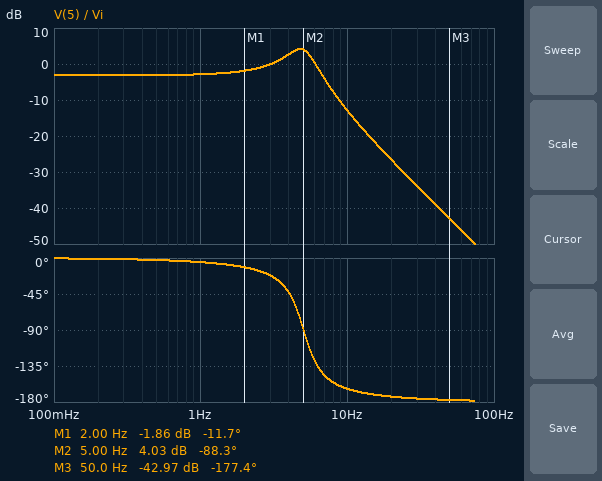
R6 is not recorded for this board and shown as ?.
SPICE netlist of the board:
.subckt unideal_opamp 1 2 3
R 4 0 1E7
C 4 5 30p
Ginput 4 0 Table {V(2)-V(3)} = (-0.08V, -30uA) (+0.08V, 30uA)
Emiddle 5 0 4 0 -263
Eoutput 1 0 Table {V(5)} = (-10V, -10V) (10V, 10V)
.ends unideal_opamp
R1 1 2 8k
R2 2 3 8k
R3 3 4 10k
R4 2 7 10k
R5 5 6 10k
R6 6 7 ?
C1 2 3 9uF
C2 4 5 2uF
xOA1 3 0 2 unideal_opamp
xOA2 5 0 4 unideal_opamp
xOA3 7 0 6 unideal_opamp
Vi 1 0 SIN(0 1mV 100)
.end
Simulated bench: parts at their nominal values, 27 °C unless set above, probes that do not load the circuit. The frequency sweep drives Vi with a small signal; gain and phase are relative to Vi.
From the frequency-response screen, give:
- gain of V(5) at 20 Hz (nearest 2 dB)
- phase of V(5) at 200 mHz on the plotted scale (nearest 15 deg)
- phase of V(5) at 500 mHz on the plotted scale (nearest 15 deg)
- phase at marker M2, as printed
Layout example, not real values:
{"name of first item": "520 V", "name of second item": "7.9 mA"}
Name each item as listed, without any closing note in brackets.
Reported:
{"gain of V(5) at 20 Hz": "-26 dB", "phase of V(5) at 200 mHz on the plotted scale": "0 deg", "phase of V(5) at 500 mHz on the plotted scale": "0 deg", "phase at marker M2, as printed": "-88.3 deg"}
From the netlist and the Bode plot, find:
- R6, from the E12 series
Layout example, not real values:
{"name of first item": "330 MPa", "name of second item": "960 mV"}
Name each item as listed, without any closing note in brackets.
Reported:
{"R6, from the E12 series": "18 kΩ"}
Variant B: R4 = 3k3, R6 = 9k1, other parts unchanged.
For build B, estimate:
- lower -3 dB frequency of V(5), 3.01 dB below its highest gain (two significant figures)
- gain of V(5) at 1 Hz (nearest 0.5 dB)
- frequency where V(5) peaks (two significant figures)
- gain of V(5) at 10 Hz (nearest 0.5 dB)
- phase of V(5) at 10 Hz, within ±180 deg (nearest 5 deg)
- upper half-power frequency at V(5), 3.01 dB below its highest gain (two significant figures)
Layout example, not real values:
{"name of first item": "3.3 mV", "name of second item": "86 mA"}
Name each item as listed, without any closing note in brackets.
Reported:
{"lower -3 dB frequency of V(5), 3.01 dB below its highest gain": "4.8 Hz", "gain of V(5) at 1 Hz": "-6.5 dB", "frequency where V(5) peaks": "6.0 Hz", "gain of V(5) at 10 Hz": "-11.5 dB", "phase of V(5) at 10 Hz, within ±180 deg": "-160 deg", "upper half-power frequency at V(5), 3.01 dB below its highest gain": "7.1 Hz"}
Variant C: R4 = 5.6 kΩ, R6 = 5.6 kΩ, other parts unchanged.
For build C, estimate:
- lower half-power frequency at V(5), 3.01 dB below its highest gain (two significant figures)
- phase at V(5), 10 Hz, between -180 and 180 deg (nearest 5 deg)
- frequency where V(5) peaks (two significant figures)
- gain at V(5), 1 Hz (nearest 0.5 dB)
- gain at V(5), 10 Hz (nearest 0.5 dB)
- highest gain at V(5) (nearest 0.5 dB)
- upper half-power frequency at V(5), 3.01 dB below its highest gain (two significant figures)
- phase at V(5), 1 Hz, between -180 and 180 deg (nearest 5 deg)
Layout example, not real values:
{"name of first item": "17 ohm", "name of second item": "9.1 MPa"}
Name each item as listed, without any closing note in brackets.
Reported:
{"lower half-power frequency at V(5), 3.01 dB below its highest gain": "1.9 Hz", "phase at V(5), 10 Hz, between -180 and 180 deg": "-165 deg", "frequency where V(5) peaks": "3.4 Hz", "gain at V(5), 1 Hz": "2.5 dB", "gain at V(5), 10 Hz": "-14.0 dB", "highest gain at V(5)": "7.0 dB", "upper half-power frequency at V(5), 3.01 dB below its highest gain": "4.4 Hz", "phase at V(5), 1 Hz, between -180 and 180 deg": "-10 deg"}
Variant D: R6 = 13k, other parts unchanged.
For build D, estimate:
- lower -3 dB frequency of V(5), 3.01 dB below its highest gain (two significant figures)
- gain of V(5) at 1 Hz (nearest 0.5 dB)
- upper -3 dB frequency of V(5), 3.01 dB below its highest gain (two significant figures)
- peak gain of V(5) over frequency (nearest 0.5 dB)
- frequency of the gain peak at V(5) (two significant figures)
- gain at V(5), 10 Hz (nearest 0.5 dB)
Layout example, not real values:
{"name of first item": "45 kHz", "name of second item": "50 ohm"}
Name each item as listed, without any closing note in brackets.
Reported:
{"lower -3 dB frequency of V(5), 3.01 dB below its highest gain": "2.6 Hz", "gain of V(5) at 1 Hz": "0 dB", "upper -3 dB frequency of V(5), 3.01 dB below its highest gain": "5.0 Hz", "peak gain of V(5) over frequency": "5.5 dB", "frequency of the gain peak at V(5)": "4.0 Hz", "gain at V(5), 10 Hz": "-13.5 dB"}
